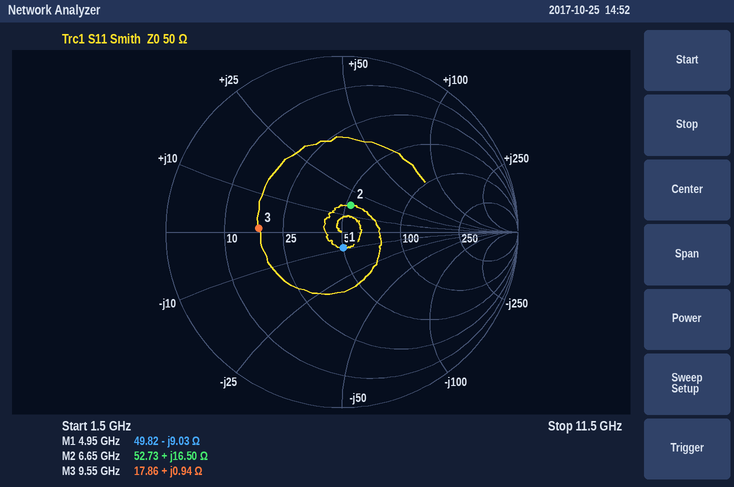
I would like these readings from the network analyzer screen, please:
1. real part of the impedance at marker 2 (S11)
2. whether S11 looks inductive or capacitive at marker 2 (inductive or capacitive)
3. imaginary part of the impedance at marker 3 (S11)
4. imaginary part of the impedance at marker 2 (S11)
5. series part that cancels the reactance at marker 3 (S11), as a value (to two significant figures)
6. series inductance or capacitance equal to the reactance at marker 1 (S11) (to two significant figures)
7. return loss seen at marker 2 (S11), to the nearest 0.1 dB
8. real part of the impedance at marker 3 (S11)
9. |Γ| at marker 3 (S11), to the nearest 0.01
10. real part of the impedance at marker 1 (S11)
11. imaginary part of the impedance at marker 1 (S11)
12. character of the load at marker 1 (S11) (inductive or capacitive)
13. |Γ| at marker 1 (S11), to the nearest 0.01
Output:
52.73 Ω
inductive
+0.94 Ω
+16.50 Ω
18 pF
3.6 pF
15.9 dB
17.86 Ω
0.47
49.82 Ω
-9.03 Ω
capacitive
0.09
